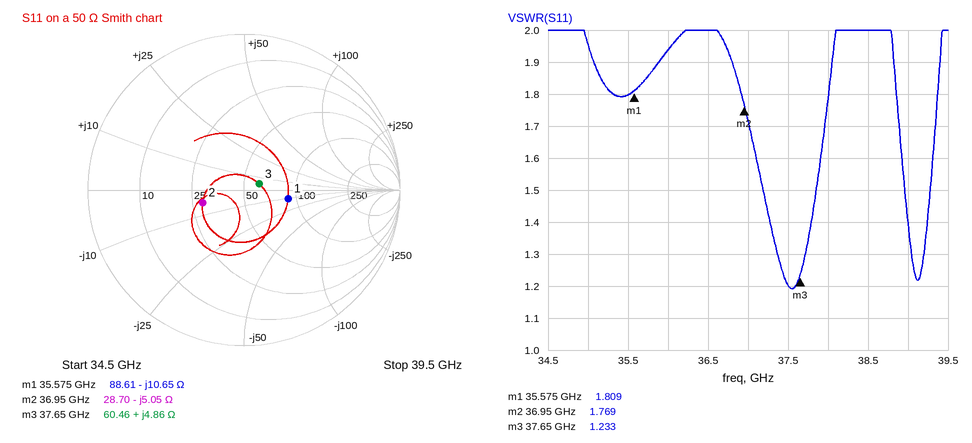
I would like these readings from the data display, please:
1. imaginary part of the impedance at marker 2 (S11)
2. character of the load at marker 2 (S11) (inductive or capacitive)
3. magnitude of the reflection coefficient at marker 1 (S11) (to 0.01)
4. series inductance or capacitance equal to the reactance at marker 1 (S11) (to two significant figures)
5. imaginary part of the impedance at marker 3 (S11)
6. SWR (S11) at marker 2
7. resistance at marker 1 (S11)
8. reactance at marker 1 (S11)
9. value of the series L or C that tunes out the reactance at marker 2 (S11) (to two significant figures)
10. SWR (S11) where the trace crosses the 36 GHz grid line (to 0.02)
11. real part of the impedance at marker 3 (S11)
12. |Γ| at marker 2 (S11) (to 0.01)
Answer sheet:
-5.05 Ω
capacitive
0.29
420 fF
+4.86 Ω
1.769
88.61 Ω
-10.65 Ω
22 pH
1.94
60.46 Ω
0.28
